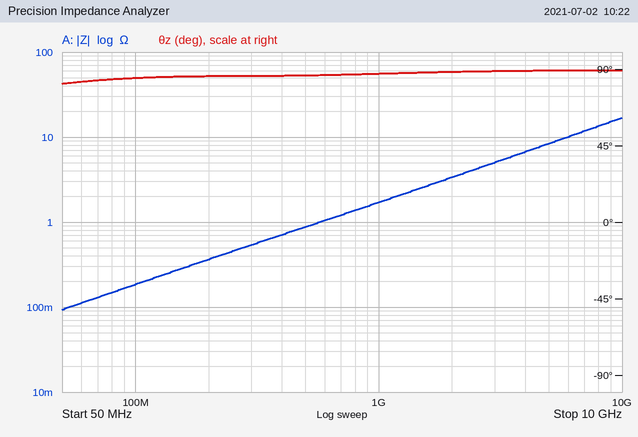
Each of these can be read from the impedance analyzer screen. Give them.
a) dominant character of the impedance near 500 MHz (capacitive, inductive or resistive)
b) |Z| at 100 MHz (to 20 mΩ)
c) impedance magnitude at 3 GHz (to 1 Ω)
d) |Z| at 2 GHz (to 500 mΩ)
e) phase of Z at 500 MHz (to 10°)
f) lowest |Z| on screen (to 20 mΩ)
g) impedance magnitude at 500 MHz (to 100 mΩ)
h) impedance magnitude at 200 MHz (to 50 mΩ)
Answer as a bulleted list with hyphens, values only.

- inductive
- 180 mΩ
- 5 Ω
- 3.5 Ω
- 90°
- 100 mΩ
- 900 mΩ
- 350 mΩ
